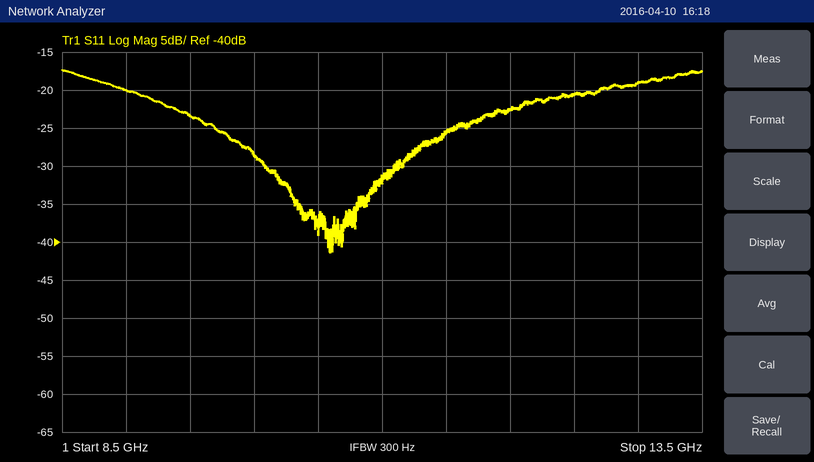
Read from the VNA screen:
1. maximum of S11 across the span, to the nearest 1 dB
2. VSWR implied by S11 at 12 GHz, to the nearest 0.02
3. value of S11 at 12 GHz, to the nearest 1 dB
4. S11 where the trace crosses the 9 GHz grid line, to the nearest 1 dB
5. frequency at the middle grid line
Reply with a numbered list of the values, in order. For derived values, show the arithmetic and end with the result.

1. -17 dB
2. |Γ| = 10^(-23/20) = 0.0708; VSWR = (1 + 0.0708)/(1 − 0.0708) ≈ 1.15, so 1.16 to the nearest 0.02
3. -23 dB
4. -20 dB
5. 11 GHz
